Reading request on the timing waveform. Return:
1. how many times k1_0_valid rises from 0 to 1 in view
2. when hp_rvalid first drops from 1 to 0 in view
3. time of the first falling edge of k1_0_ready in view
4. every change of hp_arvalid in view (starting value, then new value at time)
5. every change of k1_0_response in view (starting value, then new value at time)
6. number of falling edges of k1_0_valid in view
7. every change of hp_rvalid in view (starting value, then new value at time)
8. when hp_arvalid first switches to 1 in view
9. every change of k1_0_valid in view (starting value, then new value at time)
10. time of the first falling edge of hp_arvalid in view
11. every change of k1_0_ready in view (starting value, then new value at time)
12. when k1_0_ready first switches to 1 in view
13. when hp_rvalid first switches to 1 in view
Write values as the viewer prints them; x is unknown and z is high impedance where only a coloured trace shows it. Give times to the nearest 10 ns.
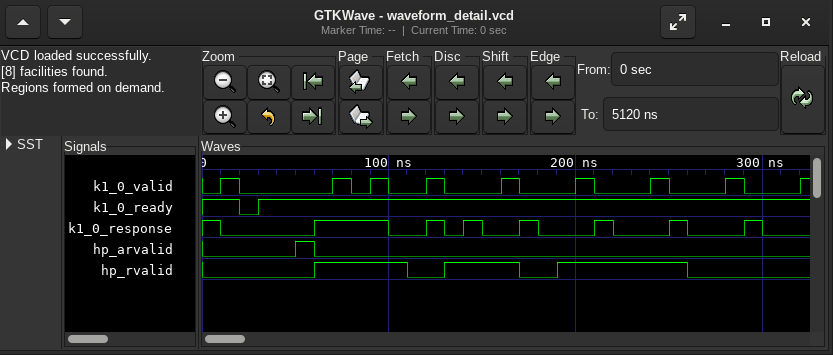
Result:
9
110 ns
20 ns
0, 1 at 50 ns, 0 at 60 ns
1, 0 at 10 ns, 1 at 60 ns, 0 at 100 ns, 1 at 120 ns, 0 at 130 ns, 1 at 140 ns, 0 at 150 ns, 1 at 170 ns, 0 at 180 ns, 1 at 210 ns, 0 at 220 ns, 1 at 250 ns, 0 at 260 ns, 1 at 290 ns, 0 at 300 ns
8
0, 1 at 60 ns, 0 at 110 ns, 1 at 130 ns, 0 at 170 ns, 1 at 190 ns, 0 at 260 ns
50 ns
0, 1 at 10 ns, 0 at 20 ns, 1 at 70 ns, 0 at 80 ns, 1 at 90 ns, 0 at 100 ns, 1 at 120 ns, 0 at 130 ns, 1 at 160 ns, 0 at 170 ns, 1 at 200 ns, 0 at 210 ns, 1 at 240 ns, 0 at 250 ns, 1 at 280 ns, 0 at 290 ns, 1 at 320 ns
60 ns
1, 0 at 20 ns, 1 at 30 ns
30 ns
60 ns
